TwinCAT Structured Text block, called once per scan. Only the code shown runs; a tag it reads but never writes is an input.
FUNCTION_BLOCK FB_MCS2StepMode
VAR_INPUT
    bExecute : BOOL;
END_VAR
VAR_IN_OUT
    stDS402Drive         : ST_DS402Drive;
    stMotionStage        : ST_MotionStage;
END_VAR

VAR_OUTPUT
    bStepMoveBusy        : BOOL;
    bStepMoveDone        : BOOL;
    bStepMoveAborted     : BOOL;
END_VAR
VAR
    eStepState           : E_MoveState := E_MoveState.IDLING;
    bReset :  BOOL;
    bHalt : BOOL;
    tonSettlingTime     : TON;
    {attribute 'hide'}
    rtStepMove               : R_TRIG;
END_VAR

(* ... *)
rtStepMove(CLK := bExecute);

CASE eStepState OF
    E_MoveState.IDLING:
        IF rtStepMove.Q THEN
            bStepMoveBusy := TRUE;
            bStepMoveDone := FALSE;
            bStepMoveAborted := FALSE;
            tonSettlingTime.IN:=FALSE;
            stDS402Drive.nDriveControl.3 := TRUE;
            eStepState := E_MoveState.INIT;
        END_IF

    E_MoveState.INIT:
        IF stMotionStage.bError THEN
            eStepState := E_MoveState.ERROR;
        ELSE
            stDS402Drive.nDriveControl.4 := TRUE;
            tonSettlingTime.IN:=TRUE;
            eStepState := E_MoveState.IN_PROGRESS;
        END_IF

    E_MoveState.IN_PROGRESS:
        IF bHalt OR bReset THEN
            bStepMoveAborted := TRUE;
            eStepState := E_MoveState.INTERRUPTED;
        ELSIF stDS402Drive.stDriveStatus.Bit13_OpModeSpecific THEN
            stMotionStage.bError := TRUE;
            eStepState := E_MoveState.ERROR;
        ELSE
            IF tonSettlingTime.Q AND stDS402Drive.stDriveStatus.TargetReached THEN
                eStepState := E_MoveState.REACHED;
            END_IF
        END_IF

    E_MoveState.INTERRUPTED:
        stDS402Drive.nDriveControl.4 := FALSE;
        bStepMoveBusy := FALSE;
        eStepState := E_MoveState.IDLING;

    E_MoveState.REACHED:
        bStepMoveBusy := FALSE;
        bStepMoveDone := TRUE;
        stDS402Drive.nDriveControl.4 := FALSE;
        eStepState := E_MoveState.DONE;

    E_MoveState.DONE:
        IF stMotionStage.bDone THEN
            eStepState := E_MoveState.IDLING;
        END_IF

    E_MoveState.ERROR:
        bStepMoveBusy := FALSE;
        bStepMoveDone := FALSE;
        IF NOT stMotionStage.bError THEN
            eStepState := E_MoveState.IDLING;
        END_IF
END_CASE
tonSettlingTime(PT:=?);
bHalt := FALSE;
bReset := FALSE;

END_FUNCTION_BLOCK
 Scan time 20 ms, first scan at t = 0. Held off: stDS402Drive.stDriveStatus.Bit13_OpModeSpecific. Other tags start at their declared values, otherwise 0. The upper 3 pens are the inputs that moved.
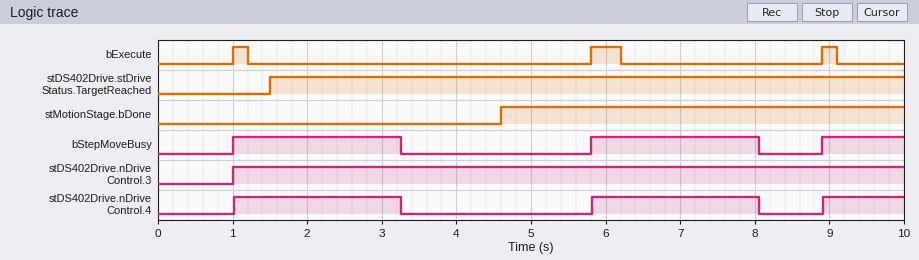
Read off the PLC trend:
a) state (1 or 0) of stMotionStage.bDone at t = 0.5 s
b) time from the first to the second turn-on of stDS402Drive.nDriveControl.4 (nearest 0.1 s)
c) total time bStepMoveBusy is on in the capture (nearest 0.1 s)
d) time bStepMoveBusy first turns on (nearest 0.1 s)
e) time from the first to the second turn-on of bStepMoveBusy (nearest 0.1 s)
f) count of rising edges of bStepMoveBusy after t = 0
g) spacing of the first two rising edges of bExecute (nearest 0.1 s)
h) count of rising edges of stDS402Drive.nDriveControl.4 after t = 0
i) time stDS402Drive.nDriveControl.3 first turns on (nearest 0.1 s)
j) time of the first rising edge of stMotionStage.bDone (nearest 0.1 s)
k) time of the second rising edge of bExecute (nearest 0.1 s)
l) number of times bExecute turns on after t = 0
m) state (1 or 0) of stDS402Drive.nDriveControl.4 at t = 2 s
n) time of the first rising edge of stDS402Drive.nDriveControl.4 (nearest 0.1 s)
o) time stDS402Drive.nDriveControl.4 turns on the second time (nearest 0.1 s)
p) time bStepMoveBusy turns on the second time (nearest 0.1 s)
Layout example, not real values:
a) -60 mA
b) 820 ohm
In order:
a) 0
b) 4.8 s
c) 5.6 s
d) 1.0 s
e) 4.8 s
f) 3
g) 4.8 s
h) 3
i) 1.0 s
j) 4.6 s
k) 5.8 s
l) 3
m) 1
n) 1.0 s
o) 5.8 s
p) 5.8 s
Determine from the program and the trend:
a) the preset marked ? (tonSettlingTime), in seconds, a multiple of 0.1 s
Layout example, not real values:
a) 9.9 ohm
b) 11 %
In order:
a) 2.2 s
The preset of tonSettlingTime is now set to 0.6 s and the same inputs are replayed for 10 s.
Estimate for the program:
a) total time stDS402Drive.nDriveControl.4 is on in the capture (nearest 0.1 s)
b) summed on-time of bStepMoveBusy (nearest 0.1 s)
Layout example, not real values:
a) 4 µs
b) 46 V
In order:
a) 1.9 s
b) 2.0 s
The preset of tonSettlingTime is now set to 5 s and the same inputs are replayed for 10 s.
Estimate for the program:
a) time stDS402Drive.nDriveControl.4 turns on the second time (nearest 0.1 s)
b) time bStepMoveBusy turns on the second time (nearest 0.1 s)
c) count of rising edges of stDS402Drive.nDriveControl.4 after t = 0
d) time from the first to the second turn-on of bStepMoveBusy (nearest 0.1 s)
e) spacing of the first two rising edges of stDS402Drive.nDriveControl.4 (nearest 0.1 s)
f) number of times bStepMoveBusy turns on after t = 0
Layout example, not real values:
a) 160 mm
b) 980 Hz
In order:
a) 8.9 s
b) 8.9 s
c) 2
d) 7.9 s
e) 7.9 s
f) 2
